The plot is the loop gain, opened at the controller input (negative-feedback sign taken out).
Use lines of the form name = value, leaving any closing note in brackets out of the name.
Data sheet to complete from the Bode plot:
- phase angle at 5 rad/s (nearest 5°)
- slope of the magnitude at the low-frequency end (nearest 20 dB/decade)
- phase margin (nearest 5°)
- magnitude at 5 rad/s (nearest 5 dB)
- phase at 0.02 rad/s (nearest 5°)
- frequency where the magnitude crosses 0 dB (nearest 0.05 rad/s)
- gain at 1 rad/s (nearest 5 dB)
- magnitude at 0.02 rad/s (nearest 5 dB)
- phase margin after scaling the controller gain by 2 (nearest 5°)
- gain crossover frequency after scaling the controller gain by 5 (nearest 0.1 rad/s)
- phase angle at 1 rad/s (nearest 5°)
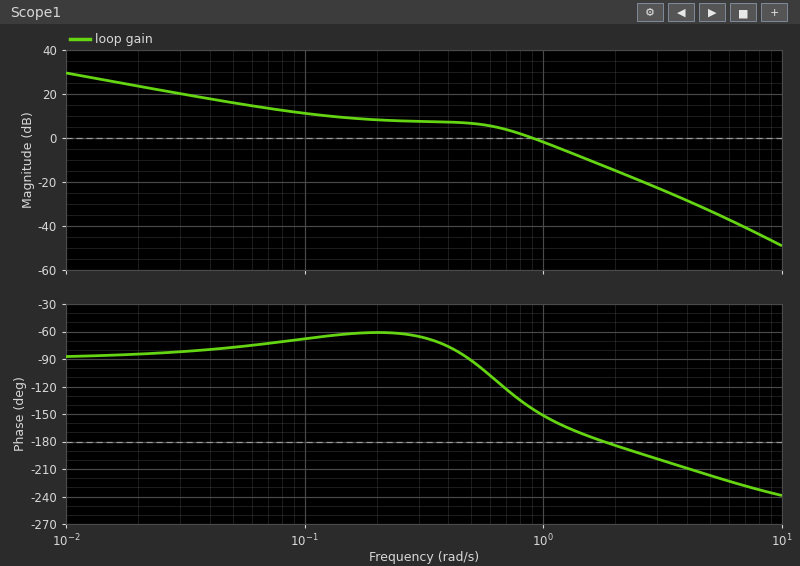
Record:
phase angle at 5 rad/s = -215°
slope of the magnitude at the low-frequency end = -20 dB/decade
phase margin = 35°
magnitude at 5 rad/s = -35 dB
phase at 0.02 rad/s = -85°
frequency where the magnitude crosses 0 dB = 0.90 rad/s
gain at 1 rad/s = 0 dB
magnitude at 0.02 rad/s = 25 dB
phase margin after scaling the controller gain by 2 = 15°
gain crossover frequency after scaling the controller gain by 5 = 1.9 rad/s
phase angle at 1 rad/s = -150°
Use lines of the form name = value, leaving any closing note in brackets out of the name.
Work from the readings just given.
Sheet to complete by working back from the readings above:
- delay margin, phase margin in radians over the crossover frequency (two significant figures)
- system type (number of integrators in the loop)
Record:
delay margin, phase margin in radians over the crossover frequency = 0.68 s
system type = 1
